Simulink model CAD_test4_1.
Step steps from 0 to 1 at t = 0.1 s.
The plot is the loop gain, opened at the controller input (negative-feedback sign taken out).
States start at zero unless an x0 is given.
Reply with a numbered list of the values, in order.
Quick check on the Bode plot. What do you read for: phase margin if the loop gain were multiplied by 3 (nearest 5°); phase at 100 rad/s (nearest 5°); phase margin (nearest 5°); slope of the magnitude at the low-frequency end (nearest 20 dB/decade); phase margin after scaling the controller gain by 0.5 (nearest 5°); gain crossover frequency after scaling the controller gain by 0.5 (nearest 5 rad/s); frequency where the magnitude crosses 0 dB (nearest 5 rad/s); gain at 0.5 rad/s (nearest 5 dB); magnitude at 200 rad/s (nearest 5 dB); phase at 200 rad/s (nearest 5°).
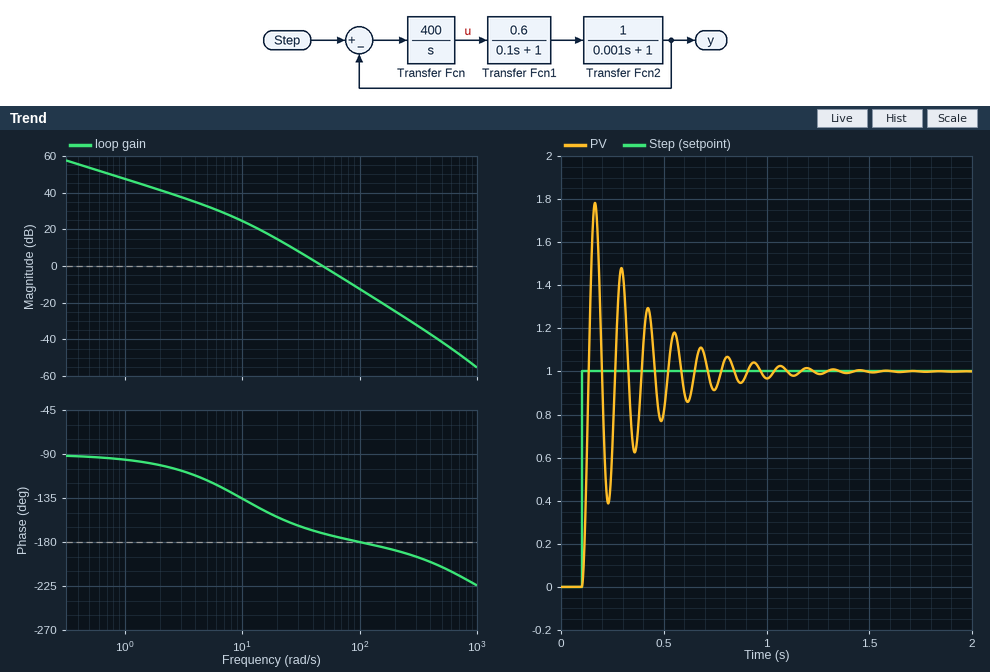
1. 0°
2. -180°
3. 10°
4. -20 dB/decade
5. 15°
6. 35 rad/s
7. 50 rad/s
8. 55 dB
9. -25 dB
10. -190°
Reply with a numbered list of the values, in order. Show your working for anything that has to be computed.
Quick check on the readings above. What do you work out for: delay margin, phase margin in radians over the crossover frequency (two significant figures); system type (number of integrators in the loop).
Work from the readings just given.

1. 10 × π / 180 / 50 = 0.0035 s
2. 1
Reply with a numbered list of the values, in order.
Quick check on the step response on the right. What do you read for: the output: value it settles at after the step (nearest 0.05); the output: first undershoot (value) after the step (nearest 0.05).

1. 1.00
2. 0.40
